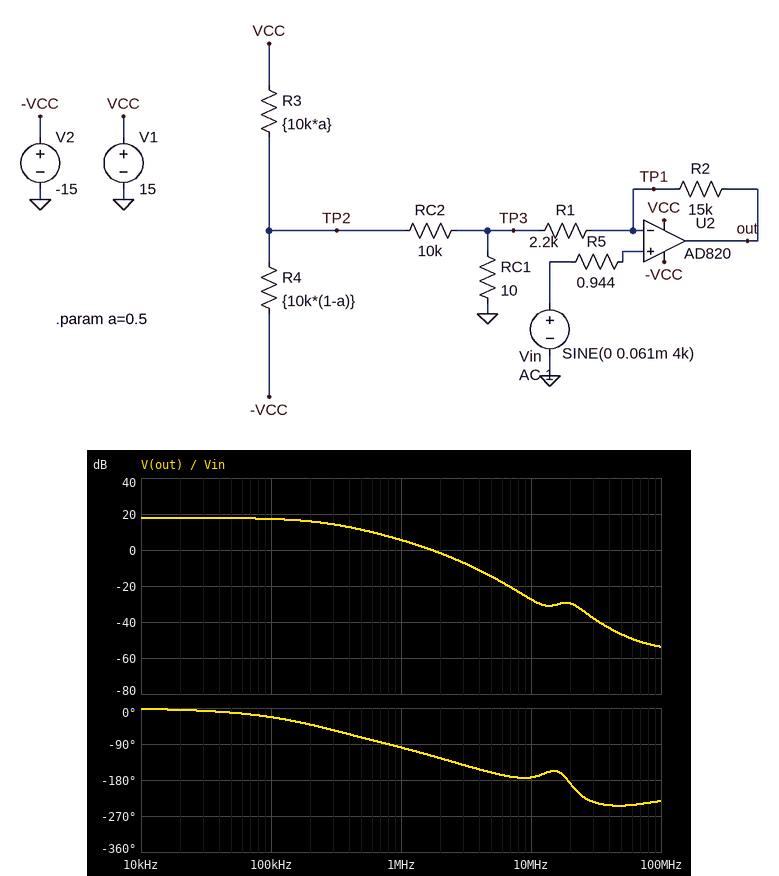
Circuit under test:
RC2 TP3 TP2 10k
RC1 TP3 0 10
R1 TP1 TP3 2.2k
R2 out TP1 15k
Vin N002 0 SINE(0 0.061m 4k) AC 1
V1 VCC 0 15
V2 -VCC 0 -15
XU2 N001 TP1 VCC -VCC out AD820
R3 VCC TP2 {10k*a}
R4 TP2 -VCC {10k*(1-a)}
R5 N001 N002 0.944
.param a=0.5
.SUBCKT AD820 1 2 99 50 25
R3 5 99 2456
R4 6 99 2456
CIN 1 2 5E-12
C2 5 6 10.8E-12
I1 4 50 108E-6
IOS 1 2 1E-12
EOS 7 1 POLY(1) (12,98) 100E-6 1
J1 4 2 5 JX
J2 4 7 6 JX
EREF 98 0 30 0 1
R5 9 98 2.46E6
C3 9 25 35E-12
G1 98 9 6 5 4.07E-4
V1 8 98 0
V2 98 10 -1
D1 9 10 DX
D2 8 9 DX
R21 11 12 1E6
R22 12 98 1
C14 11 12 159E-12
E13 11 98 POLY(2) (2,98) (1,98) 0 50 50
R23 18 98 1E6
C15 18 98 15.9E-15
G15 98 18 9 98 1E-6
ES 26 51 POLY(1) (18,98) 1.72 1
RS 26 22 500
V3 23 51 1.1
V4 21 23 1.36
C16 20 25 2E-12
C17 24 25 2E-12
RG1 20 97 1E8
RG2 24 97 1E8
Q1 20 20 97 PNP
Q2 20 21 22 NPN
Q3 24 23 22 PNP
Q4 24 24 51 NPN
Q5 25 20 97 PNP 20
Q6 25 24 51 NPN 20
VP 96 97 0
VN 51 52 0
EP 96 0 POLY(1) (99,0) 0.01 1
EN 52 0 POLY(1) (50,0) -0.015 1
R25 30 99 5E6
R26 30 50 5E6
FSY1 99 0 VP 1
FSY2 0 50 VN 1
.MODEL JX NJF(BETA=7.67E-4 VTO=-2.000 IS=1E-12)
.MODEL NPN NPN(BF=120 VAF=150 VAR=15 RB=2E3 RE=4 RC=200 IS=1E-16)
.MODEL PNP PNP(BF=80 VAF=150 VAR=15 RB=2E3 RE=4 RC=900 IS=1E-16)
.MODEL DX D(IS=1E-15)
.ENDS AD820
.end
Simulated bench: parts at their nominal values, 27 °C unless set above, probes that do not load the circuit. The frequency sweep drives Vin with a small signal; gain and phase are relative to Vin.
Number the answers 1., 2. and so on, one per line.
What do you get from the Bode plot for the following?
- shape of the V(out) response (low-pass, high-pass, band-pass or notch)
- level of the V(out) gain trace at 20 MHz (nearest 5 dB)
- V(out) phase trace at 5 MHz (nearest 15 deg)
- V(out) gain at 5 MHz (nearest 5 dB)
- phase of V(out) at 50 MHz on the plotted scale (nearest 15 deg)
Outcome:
1. low-pass
2. -30 dB
3. -165 deg
4. -15 dB
5. -240 deg
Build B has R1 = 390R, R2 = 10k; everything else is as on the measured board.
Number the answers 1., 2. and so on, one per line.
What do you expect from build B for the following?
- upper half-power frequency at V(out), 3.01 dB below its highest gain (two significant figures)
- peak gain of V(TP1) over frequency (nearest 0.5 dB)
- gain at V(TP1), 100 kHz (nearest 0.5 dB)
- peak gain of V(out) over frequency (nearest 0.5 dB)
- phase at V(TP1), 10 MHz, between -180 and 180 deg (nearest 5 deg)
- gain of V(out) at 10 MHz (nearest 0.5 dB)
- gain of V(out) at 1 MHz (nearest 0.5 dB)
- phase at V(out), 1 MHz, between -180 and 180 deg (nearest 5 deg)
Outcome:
1. 73 kHz
2. 0 dB
3. -4.5 dB
4. 28.5 dB
5. 85 deg
6. -22.0 dB
7. 5.0 dB
8. -105 deg
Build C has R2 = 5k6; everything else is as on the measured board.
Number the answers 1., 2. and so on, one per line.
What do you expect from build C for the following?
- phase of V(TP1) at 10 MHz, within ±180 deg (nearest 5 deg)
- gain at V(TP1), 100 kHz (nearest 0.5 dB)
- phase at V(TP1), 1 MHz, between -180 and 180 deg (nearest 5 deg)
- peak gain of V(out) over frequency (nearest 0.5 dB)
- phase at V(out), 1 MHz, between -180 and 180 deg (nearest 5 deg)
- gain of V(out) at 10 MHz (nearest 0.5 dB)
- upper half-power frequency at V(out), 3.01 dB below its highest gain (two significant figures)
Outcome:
1. 65 deg
2. 0 dB
3. -85 deg
4. 11.0 dB
5. -80 deg
6. -26.0 dB
7. 690 kHz
